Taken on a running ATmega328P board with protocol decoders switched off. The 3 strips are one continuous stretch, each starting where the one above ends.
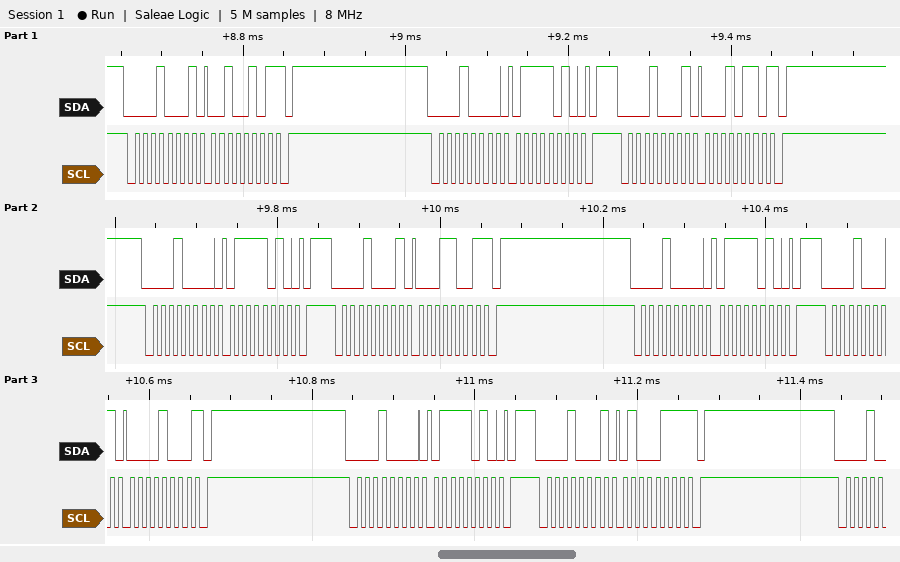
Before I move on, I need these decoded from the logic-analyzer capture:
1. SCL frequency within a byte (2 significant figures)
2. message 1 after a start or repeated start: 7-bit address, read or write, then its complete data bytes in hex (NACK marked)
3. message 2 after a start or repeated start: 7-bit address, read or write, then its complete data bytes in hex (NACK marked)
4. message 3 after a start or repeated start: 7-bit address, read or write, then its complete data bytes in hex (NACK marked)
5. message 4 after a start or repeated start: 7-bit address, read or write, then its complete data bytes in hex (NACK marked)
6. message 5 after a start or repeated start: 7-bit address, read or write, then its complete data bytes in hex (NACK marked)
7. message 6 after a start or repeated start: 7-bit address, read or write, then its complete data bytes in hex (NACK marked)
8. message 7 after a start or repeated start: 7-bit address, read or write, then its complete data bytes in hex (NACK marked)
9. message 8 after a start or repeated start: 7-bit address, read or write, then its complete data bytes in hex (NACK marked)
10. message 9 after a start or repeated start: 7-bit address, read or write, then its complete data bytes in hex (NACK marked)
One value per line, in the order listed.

100 kHz
0x08 read: 25 NACK
0x08 write: 7A
0x08 read: 16 NACK
0x08 write: 7A
0x08 read: 19 NACK
0x08 write: 7A
0x08 read: 08 NACK
0x08 write: 7A
0x08 read: 47 NACK
